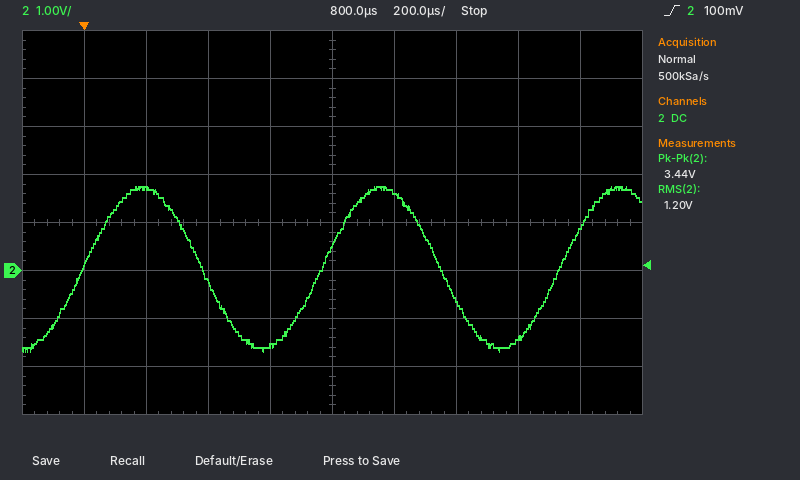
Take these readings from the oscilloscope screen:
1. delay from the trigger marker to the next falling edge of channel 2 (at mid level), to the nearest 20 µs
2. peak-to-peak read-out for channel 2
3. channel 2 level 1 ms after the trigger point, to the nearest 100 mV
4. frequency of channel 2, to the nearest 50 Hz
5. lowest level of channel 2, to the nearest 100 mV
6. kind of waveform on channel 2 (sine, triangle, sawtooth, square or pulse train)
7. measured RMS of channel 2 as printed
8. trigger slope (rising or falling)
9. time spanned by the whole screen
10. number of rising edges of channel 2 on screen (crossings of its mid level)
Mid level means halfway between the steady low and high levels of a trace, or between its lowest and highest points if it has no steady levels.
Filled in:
380 µs
3.44 V
1.6 V
1.30 kHz
-1.7 V
sine
1.20 V
rising
2 ms
3
